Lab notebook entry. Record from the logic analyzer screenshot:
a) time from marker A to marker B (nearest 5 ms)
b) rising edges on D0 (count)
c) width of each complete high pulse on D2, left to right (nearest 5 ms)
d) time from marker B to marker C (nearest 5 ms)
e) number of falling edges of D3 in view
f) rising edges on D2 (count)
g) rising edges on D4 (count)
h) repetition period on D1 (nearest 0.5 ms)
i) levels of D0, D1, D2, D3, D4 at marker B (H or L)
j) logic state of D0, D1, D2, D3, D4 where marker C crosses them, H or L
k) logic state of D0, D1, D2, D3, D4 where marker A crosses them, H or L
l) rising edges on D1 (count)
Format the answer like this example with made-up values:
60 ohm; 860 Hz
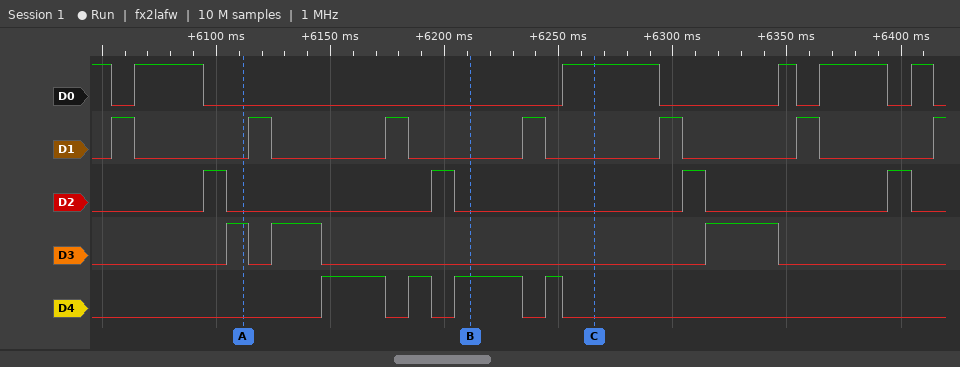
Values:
100 ms; 5; 10 ms, 10 ms, 10 ms, 10 ms; 55 ms; 3; 4; 4; 60 ms; D0=L, D1=L, D2=L, D3=L, D4=H; D0=H, D1=L, D2=L, D3=L, D4=L; D0=L, D1=L, D2=L, D3=H, D4=L; 7
